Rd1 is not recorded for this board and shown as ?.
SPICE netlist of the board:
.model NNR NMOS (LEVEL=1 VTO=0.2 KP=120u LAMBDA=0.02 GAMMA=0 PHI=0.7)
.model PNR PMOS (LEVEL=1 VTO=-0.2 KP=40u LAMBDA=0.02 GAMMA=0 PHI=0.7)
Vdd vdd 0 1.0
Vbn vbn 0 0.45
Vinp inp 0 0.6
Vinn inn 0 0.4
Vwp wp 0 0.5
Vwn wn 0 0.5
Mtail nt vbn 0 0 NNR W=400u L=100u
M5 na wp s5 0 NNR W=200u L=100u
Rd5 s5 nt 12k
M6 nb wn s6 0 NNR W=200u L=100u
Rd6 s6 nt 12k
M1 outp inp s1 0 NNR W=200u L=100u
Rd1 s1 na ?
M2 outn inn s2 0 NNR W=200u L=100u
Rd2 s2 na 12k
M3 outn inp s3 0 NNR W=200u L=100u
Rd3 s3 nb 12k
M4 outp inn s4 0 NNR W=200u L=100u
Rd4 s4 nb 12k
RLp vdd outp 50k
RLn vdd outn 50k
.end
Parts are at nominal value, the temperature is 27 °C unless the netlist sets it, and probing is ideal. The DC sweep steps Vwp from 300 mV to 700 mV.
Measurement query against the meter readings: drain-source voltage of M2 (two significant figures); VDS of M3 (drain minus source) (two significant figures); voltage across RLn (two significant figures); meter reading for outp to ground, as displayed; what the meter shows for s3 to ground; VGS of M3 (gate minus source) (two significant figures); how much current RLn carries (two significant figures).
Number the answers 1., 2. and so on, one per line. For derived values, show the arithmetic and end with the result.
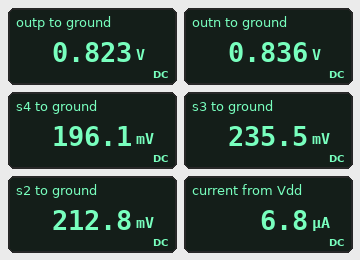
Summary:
1. 836 mV - 212.8 mV = 620 mV
2. 836 mV - 235.5 mV = 600 mV
3. 1 V - 836 mV = 160 mV
4. 0.823 V
5. 235.5 mV
6. 600 mV - 235.5 mV = 360 mV
7. (1 V - 836 mV) / 50 kΩ = 3.3 µA
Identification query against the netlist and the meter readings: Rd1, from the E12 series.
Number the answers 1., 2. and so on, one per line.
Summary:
1. 4.7 kΩ
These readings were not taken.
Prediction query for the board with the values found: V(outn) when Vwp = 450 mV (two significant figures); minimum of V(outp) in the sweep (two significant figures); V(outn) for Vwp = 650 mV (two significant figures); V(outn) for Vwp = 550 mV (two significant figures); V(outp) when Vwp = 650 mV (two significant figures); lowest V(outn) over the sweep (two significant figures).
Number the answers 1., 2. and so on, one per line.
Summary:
1. 830 mV
2. 770 mV
3. 840 mV
4. 840 mV
5. 780 mV
6. 810 mV
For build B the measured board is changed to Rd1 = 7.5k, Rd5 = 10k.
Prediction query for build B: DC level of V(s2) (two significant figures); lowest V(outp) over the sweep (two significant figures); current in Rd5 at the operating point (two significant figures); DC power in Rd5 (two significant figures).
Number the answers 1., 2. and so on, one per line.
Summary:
1. 200 mV
2. 780 mV
3. 3.6 µA
4. 130 nW
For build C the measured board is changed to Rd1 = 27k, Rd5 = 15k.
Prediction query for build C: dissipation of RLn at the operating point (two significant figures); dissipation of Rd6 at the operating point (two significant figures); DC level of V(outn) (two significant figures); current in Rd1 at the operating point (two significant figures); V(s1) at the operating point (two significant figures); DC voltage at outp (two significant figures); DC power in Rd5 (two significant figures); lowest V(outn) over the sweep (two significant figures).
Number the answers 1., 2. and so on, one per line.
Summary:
1. 600 nW
2. 140 nW
3. 830 mV
4. 2.8 µA
5. 250 mV
6. 860 mV
7. 120 nW
8. 810 mV
